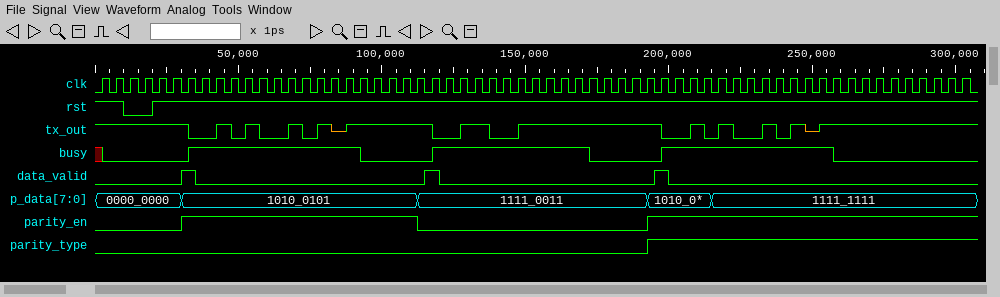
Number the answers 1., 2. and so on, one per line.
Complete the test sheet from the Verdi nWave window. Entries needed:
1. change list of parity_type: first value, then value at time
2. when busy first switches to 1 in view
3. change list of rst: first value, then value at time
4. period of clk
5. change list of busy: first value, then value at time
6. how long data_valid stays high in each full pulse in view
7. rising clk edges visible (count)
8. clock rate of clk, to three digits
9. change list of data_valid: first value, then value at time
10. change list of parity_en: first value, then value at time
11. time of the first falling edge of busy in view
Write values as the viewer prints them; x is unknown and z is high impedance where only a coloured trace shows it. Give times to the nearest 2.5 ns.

1. 0, 1 at 192.5 ns
2. 32.5 ns
3. 1, 0 at 10 ns, 1 at 20 ns
4. 5 ns
5. x, 0 at 2.5 ns, 1 at 32.5 ns, 0 at 92.5 ns, 1 at 117.5 ns, 0 at 172.5 ns, 1 at 197.5 ns, 0 at 257.5 ns
6. 5 ns, 5 ns, 5 ns
7. 61
8. 200 MHz
9. 0, 1 at 30 ns, 0 at 35 ns, 1 at 115 ns, 0 at 120 ns, 1 at 195 ns, 0 at 200 ns
10. 0, 1 at 30 ns, 0 at 112.5 ns, 1 at 192.5 ns
11. 92.5 ns
